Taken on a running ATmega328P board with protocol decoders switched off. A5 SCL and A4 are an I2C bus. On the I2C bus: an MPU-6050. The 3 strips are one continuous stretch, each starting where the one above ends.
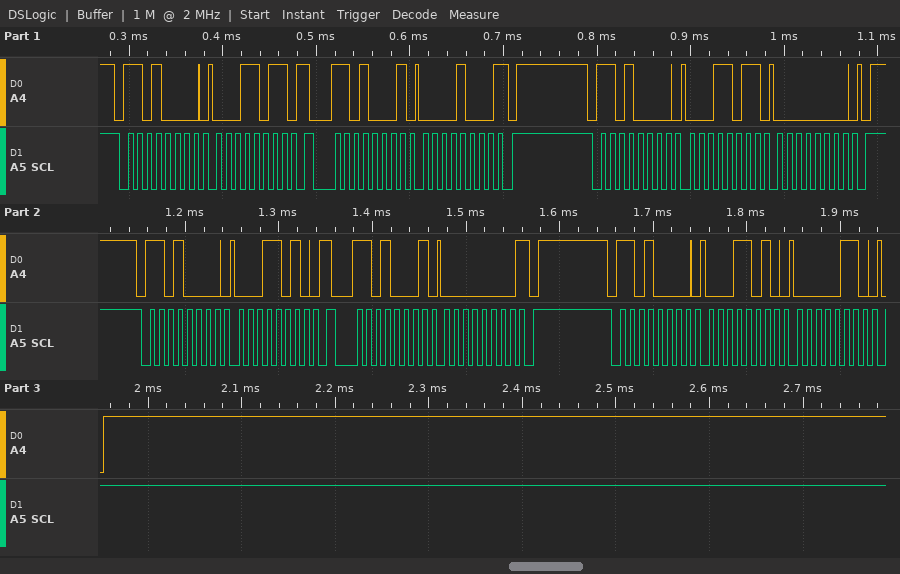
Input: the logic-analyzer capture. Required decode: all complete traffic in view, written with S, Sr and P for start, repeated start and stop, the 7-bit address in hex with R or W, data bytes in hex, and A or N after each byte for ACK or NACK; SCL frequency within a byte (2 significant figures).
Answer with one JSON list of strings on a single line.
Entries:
["S 68W A 1B A Sr 68R A 08 N P S 68W A 1B A 00 A P S 68W A 1A A Sr 68R A 00 N P S 68W A 1A A 06 A P", "100 kHz"]
